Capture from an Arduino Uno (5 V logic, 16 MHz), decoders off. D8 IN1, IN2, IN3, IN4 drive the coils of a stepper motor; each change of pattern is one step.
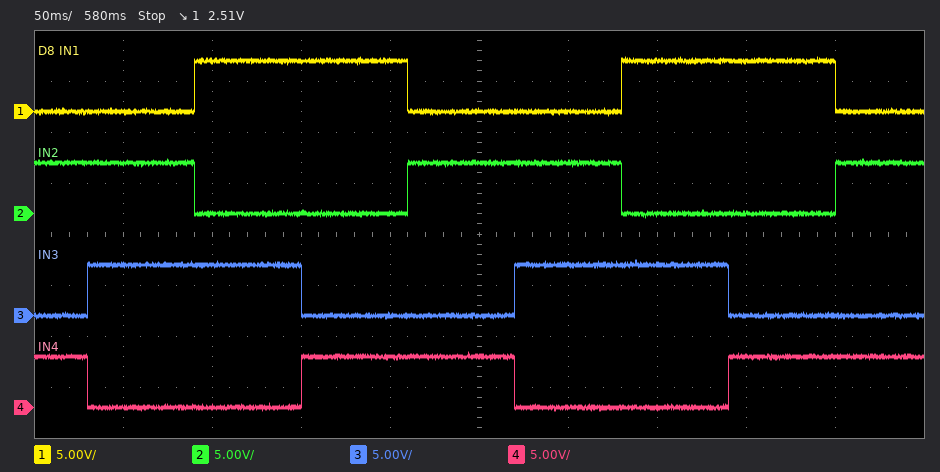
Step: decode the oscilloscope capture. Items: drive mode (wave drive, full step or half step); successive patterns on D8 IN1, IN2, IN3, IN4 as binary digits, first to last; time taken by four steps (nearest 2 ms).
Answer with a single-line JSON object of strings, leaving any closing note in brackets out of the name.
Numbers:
{"drive mode": "full step", "successive patterns on D8 IN1, IN2, IN3, IN4 as binary digits, first to last": "0101 0110 1010 1001 0101 0110 1010 1001 0101", "time taken by four steps": "240 ms"}
